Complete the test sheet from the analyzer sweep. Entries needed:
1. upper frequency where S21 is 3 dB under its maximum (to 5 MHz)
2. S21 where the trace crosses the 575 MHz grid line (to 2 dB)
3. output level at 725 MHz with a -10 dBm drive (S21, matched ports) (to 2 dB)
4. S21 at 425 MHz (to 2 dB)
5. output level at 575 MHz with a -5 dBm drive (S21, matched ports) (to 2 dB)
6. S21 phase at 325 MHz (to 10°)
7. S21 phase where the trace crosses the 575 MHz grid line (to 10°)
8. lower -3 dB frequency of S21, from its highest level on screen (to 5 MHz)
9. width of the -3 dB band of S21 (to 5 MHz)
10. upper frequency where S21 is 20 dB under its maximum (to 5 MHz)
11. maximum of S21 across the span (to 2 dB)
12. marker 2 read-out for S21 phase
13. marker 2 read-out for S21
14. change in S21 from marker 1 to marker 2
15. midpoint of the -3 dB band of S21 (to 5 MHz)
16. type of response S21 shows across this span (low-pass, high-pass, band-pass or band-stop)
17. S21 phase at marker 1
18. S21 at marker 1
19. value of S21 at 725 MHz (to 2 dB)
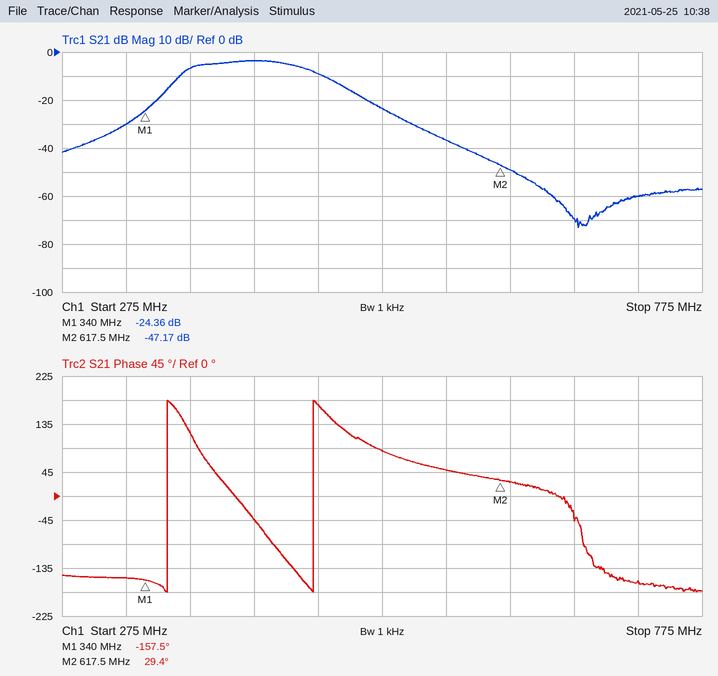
465 MHz
-36 dB
-70 dBm
-4 dB
-42 dBm
-150°
50°
375 MHz
90 MHz
525 MHz
-4 dB
29.4°
-47.17 dB
-22.81 dB
420 MHz
band-pass
-157.5°
-24.36 dB
-60 dB
